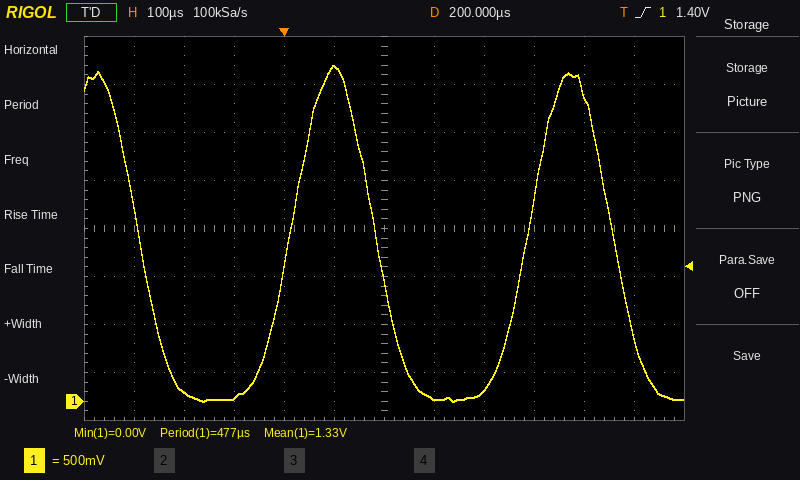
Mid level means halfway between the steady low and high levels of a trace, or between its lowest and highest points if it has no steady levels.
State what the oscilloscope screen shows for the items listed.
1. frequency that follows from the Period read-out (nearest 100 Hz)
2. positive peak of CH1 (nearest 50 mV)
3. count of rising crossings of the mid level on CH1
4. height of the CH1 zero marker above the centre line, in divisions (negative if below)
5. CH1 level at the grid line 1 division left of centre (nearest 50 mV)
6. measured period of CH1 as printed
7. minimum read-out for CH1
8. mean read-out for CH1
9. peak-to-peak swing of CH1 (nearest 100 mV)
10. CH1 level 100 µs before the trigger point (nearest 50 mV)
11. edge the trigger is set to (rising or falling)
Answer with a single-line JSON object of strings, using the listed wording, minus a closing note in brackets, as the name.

{"frequency that follows from the Period read-out": "2.1 kHz", "positive peak of CH1": "3.50 V", "count of rising crossings of the mid level on CH1": "2", "height of the CH1 zero marker above the centre line, in divisions": "-3.6 div", "CH1 level at the grid line 1 division left of centre": "3.50 V", "measured period of CH1 as printed": "477 µs", "minimum read-out for CH1": "0.00 V", "mean read-out for CH1": "1.33 V", "peak-to-peak swing of CH1": "3.50 V", "CH1 level 100 µs before the trigger point": "50 mV", "edge the trigger is set to": "rising"}
